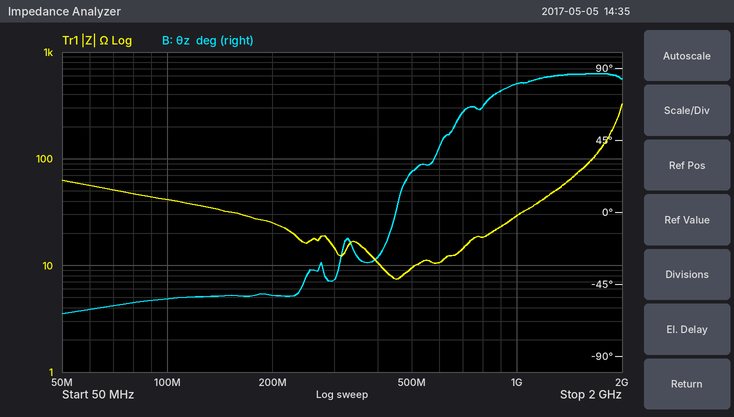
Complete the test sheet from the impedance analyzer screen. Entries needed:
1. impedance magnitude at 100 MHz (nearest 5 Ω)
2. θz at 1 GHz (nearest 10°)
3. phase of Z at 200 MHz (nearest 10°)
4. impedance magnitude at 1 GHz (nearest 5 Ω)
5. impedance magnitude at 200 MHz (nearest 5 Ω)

40 Ω
80°
-50°
30 Ω
25 Ω
